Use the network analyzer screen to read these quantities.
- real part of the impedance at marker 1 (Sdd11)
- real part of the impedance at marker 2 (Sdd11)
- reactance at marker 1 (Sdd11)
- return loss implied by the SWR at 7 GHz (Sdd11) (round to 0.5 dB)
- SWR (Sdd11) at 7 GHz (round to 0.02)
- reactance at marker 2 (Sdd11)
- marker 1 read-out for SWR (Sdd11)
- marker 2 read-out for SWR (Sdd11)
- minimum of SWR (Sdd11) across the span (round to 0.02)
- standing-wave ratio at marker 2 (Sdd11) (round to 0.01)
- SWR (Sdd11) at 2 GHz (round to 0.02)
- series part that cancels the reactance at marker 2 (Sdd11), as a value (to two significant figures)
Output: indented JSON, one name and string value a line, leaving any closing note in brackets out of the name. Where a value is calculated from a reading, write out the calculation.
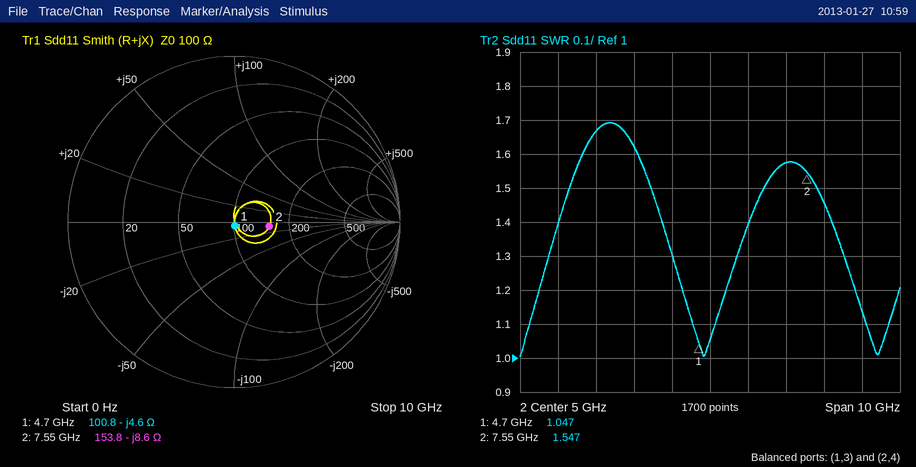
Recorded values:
{
  "real part of the impedance at marker 1": "100.8 Ω",
  "real part of the impedance at marker 2": "153.8 Ω",
  "reactance at marker 1": "-4.6 Ω",
  "return loss implied by the SWR at 7 GHz (Sdd11)": "−20 log10((1.58 − 1)/(1.58 + 1)) ≈ 13.0 dB",
  "SWR (Sdd11) at 7 GHz": "1.58",
  "reactance at marker 2": "-8.6 Ω",
  "marker 1 read-out for SWR": "1.047",
  "marker 2 read-out for SWR": "1.547",
  "minimum of SWR (Sdd11) across the span": "1.00",
  "standing-wave ratio at marker 2 (Sdd11)": "1.55",
  "SWR (Sdd11) at 2 GHz": "1.66",
  "series part that cancels the reactance at marker 2 (Sdd11), as a value": "L = 8.6 Ω/(2π × 7.55 GHz) ≈ 181 pH, so 180 pH to two significant figures"
}
